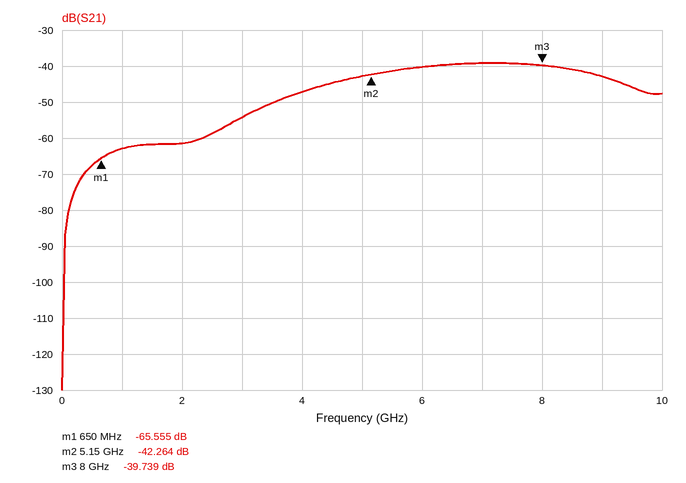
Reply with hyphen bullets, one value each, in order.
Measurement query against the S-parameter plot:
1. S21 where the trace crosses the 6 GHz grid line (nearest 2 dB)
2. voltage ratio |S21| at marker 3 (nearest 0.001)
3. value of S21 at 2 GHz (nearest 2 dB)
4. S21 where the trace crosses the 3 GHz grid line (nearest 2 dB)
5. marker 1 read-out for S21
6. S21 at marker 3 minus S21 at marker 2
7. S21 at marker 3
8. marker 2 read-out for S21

- -40 dB
- 0.010
- -62 dB
- -54 dB
- -65.555 dB
- 2.525 dB
- -39.739 dB
- -42.264 dB
